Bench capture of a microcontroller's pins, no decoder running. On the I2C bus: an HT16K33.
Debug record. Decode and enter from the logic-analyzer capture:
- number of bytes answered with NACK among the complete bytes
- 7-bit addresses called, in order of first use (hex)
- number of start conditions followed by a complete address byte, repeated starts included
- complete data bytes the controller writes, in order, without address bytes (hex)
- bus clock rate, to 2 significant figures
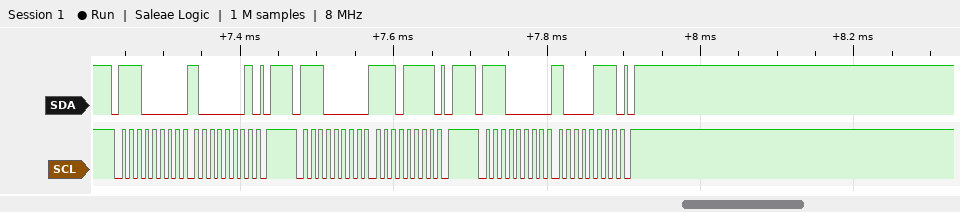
0
0x70
3
81 EF 87
100 kHz
